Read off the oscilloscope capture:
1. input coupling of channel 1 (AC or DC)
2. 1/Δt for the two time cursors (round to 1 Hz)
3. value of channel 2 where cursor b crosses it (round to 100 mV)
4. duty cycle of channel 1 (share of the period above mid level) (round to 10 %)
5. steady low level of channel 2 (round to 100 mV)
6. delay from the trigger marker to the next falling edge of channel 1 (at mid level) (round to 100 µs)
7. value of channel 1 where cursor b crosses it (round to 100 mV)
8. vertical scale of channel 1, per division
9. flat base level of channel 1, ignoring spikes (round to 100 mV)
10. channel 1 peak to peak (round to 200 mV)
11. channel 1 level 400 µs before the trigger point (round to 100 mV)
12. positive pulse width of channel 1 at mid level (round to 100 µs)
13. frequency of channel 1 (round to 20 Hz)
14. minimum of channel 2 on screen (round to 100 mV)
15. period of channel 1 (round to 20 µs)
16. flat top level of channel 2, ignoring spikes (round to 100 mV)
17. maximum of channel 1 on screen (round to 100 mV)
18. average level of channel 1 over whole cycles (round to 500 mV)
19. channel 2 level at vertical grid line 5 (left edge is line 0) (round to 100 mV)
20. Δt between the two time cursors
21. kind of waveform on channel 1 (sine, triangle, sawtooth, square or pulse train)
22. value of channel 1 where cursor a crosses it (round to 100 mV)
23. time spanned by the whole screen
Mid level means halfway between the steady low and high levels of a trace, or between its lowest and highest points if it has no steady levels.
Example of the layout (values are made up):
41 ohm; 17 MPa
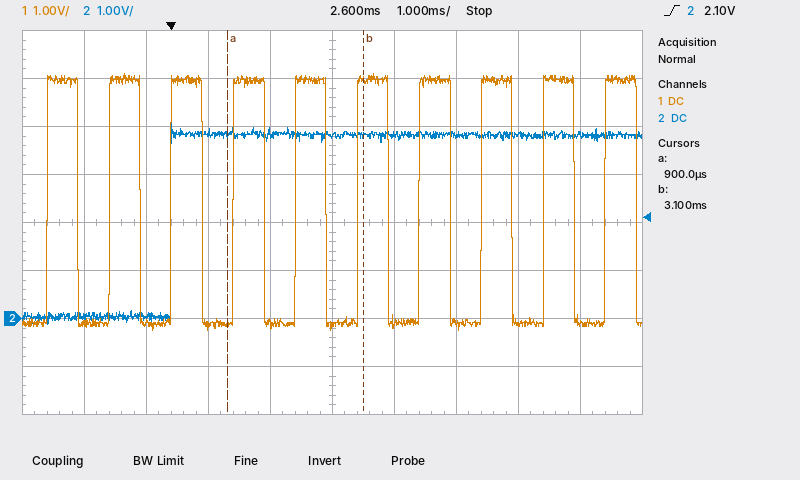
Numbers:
DC; 455 Hz; 3.8 V; 50 %; 0.0 V; 500 µs; 5.0 V; 1 V; -100 mV; 5.4 V; -100 mV; 500 µs; 1.00 kHz; -100 mV; 1.00 ms; 3.8 V; 5.1 V; 2.5 V; 3.8 V; 2.2 ms; square; -100 mV; 10 ms
